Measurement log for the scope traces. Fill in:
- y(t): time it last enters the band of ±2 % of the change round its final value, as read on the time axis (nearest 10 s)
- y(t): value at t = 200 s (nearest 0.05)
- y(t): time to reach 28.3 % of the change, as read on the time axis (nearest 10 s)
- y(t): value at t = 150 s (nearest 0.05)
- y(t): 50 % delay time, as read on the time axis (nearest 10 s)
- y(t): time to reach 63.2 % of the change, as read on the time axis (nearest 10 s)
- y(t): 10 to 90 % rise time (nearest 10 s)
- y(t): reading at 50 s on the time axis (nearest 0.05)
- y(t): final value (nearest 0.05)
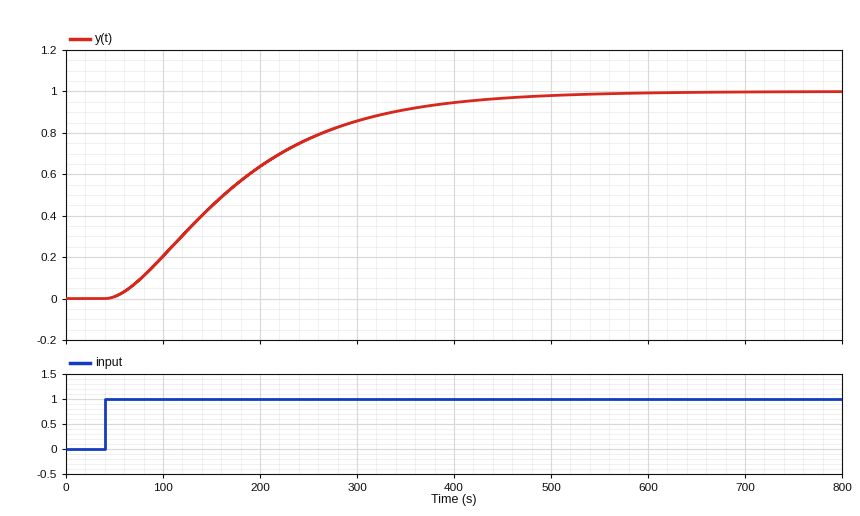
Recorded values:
500 s
0.65
120 s
0.45
160 s
200 s
260 s
0.00
1.00
